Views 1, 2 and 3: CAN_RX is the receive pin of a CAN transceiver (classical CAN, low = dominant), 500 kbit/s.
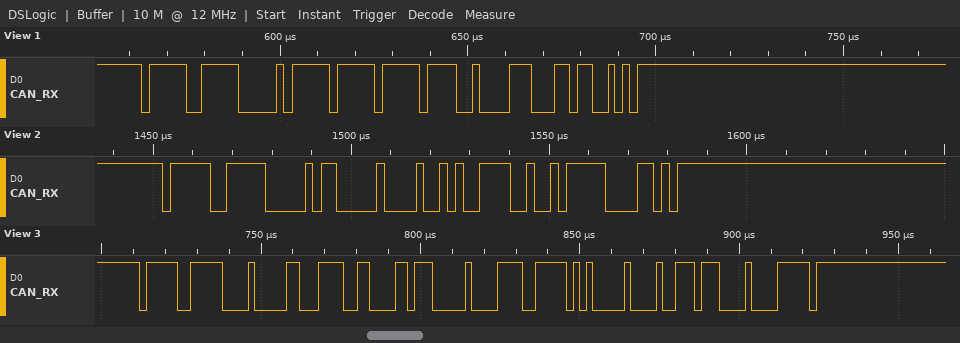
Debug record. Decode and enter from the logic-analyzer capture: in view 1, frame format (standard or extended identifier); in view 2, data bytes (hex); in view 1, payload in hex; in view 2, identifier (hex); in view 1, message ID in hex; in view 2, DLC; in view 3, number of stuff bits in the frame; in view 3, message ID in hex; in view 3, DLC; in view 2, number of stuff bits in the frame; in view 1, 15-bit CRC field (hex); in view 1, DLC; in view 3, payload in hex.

standard
00 4A 79
FF FF 90
0x7DF
0x7DF
3
6
0x7DF
8
5
0x71B2
3
23 CC 37 00 79 FA 00 9D
